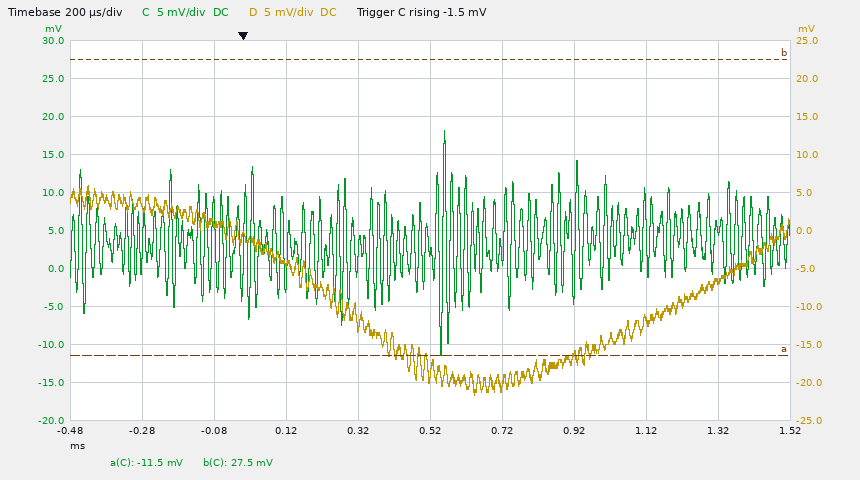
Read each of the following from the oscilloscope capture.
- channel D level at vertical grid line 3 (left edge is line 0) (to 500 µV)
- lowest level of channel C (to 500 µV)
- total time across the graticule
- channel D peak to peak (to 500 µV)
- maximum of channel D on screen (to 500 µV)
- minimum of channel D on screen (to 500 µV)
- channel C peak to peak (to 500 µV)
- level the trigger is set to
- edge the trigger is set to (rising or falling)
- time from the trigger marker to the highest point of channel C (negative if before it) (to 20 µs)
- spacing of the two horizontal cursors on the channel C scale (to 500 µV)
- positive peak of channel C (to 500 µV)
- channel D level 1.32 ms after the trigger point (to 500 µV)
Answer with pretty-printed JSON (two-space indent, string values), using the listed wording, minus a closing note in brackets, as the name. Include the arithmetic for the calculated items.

{
  "channel D level at vertical grid line 3 (left edge is line 0)": "-4.5 mV",
  "lowest level of channel C": "-11.5 mV",
  "total time across the graticule": "2 ms",
  "channel D peak to peak": "6.0 mV − (-21.5 mV) = 27.5 mV",
  "maximum of channel D on screen": "6.0 mV",
  "minimum of channel D on screen": "-21.5 mV",
  "channel C peak to peak": "18.0 mV − (-11.5 mV) = 29.5 mV",
  "level the trigger is set to": "-1.5 mV",
  "edge the trigger is set to": "rising",
  "time from the trigger marker to the highest point of channel C (negative if before it)": "+560 µs",
  "spacing of the two horizontal cursors on the channel C scale": "39.0 mV",
  "positive peak of channel C": "18.0 mV",
  "channel D level 1.32 ms after the trigger point": "-6.5 mV"
}
